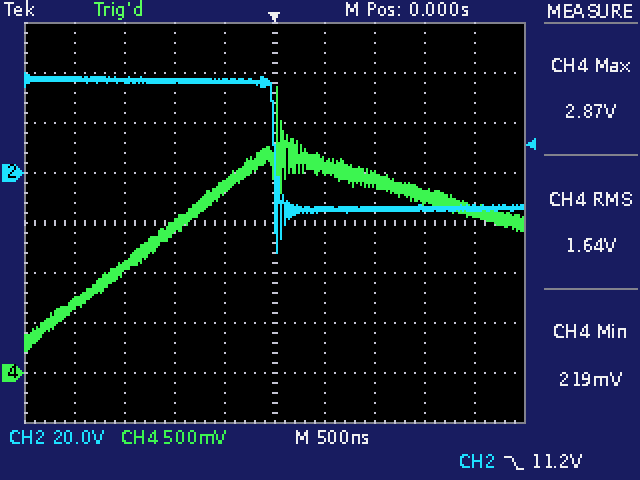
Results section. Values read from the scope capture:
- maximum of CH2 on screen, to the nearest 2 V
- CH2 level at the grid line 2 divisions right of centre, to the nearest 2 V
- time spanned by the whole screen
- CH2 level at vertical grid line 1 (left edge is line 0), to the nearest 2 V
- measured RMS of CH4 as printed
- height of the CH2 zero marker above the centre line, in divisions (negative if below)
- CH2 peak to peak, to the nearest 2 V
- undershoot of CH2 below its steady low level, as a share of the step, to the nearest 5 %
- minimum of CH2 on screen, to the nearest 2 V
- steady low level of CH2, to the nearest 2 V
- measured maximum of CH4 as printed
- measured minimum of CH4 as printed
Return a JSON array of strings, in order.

["40 V", "-14 V", "5 µs", "38 V", "1.64 V", "+1.0 div", "72 V", "35 %", "-32 V", "-14 V", "2.87 V", "219 mV"]
